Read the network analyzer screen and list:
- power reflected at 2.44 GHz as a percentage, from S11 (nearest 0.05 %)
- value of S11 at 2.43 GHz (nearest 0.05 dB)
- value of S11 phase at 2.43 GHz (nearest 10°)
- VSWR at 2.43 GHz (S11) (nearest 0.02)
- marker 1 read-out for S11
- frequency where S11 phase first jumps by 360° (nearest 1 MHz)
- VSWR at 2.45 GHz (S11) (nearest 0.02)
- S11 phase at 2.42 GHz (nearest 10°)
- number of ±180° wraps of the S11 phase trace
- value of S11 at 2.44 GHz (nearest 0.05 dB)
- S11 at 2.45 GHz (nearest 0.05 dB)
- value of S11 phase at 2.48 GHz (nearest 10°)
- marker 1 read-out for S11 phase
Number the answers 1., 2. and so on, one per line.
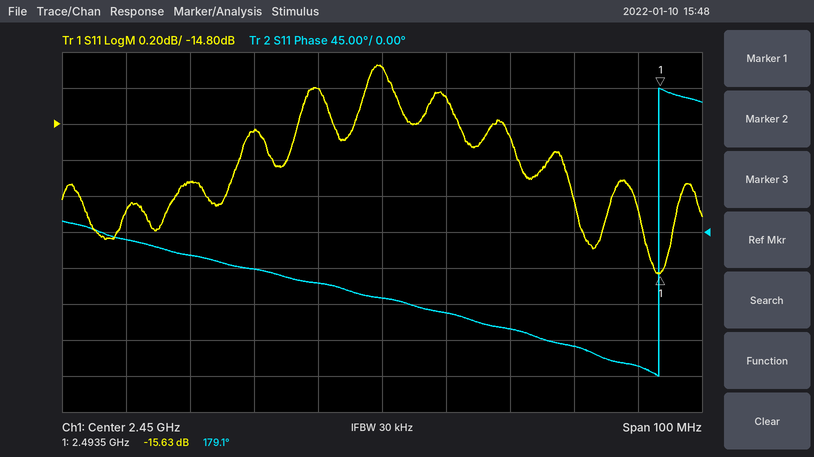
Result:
1. 3.45 %
2. -14.85 dB
3. -50°
4. 1.44
5. -15.63 dB
6. 2.493 GHz
7. 1.46
8. -30°
9. 1
10. -14.60 dB
11. -14.50 dB
12. -140°
13. 179.1°
